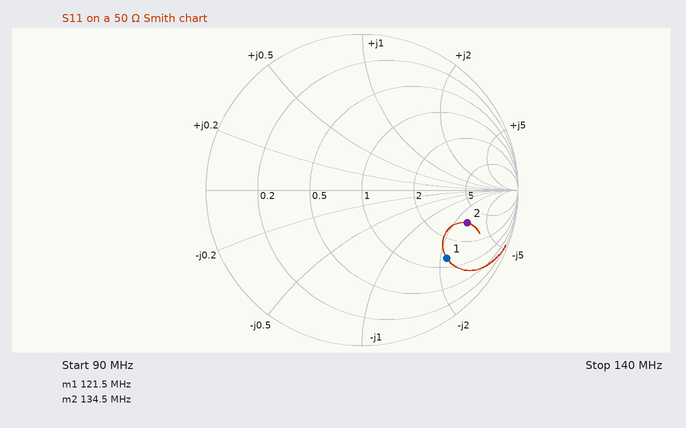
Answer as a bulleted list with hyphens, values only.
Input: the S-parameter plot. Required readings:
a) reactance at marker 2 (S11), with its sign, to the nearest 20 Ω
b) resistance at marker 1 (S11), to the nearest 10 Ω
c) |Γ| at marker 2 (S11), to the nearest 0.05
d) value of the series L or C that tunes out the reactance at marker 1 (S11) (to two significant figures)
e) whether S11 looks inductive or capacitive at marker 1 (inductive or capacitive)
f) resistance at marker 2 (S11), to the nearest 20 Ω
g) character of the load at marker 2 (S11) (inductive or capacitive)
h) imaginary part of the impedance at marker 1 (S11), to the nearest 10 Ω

- -140 Ω
- 60 Ω
- 0.70
- 140 nH
- capacitive
- 160 Ω
- capacitive
- -110 Ω
